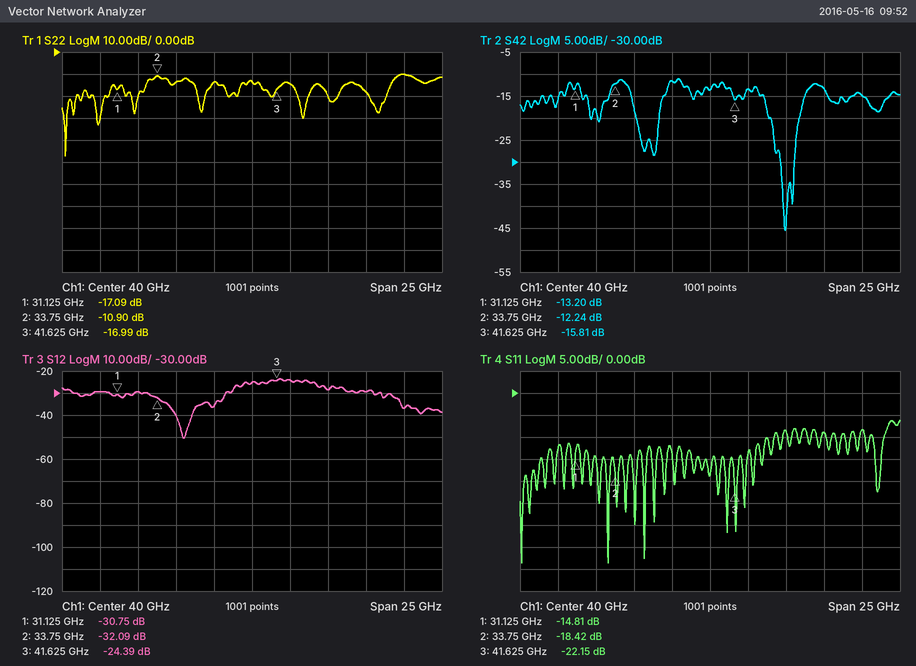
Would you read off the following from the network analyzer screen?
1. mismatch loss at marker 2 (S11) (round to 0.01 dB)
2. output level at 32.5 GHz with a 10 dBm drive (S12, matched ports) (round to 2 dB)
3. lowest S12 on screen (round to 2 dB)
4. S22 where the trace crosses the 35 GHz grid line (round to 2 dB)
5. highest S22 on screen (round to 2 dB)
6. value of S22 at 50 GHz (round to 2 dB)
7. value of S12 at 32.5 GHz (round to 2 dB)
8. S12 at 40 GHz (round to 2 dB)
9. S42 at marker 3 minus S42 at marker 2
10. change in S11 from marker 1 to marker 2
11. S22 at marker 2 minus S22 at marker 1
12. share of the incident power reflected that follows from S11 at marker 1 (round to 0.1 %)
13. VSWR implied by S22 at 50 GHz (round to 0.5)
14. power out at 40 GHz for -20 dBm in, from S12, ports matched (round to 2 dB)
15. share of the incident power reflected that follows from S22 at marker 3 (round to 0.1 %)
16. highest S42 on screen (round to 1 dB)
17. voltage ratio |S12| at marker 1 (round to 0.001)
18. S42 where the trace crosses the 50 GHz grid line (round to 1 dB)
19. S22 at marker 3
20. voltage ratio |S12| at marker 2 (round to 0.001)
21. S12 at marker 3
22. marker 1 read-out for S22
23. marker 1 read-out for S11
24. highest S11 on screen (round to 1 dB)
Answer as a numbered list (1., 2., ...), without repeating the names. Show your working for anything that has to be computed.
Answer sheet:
1. −10 log10(1 − 10^(-18.42/10)) ≈ 0.06 dB
2. 10 dBm + (-30 dB) = -20 dBm
3. -50 dB
4. -14 dB
5. -10 dB
6. -10 dB
7. -30 dB
8. -26 dB
9. -15.81 − (-12.24) = -3.57 dB
10. -18.42 − (-14.81) = -3.61 dB
11. -10.9 − (-17.09) = 6.19 dB
12. 10^(-14.81/10) ≈ 3.3 %
13. |Γ| = 10^(-10/20) = 0.3162; VSWR = (1 + 0.3162)/(1 − 0.3162) ≈ 1.92, so 2.0 to the nearest 0.5
14. -20 dBm + (-26 dB) = -46 dBm
15. 10^(-16.99/10) ≈ 2.0 %
16. -11 dB
17. 10^(-30.75/20) ≈ 0.029
18. -15 dB
19. -16.99 dB
20. 10^(-32.09/20) ≈ 0.025
21. -24.39 dB
22. -17.09 dB
23. -14.81 dB
24. -6 dB
